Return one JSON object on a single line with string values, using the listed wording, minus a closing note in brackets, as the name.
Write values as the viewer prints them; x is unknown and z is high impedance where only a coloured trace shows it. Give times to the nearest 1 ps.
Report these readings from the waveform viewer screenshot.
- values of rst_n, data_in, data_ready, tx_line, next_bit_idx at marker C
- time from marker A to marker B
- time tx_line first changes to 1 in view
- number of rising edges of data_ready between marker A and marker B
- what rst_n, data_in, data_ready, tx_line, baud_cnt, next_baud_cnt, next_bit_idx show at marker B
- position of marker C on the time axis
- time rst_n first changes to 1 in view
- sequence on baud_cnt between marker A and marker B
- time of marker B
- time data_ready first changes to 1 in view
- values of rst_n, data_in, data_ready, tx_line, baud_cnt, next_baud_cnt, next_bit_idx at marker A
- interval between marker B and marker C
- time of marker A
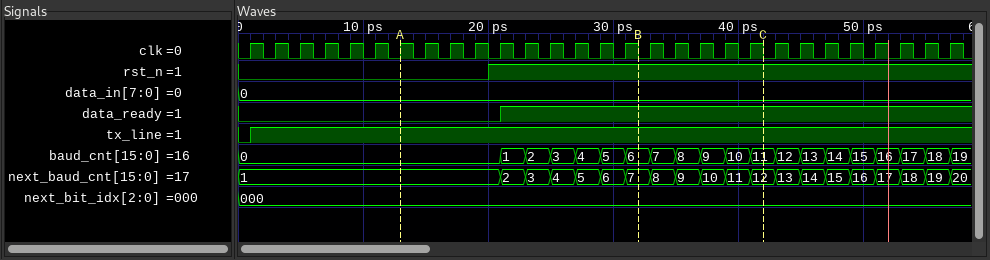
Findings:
{"values of rst_n, data_in, data_ready, tx_line, next_bit_idx at marker C": "rst_n=1, data_in=0, data_ready=1, tx_line=1, next_bit_idx=000", "time from marker A to marker B": "19 ps", "time tx_line first changes to 1 in view": "1 ps", "number of rising edges of data_ready between marker A and marker B": "1", "what rst_n, data_in, data_ready, tx_line, baud_cnt, next_baud_cnt, next_bit_idx show at marker B": "rst_n=1, data_in=0, data_ready=1, tx_line=1, baud_cnt=6, next_baud_cnt=7, next_bit_idx=000", "position of marker C on the time axis": "42 ps", "time rst_n first changes to 1 in view": "20 ps", "sequence on baud_cnt between marker A and marker B": "0, 1, 2, 3, 4, 5, 6", "time of marker B": "32 ps", "time data_ready first changes to 1 in view": "21 ps", "values of rst_n, data_in, data_ready, tx_line, baud_cnt, next_baud_cnt, next_bit_idx at marker A": "rst_n=0, data_in=0, data_ready=0, tx_line=1, baud_cnt=0, next_baud_cnt=1, next_bit_idx=000", "interval between marker B and marker C": "10 ps", "time of marker A": "13 ps"}
